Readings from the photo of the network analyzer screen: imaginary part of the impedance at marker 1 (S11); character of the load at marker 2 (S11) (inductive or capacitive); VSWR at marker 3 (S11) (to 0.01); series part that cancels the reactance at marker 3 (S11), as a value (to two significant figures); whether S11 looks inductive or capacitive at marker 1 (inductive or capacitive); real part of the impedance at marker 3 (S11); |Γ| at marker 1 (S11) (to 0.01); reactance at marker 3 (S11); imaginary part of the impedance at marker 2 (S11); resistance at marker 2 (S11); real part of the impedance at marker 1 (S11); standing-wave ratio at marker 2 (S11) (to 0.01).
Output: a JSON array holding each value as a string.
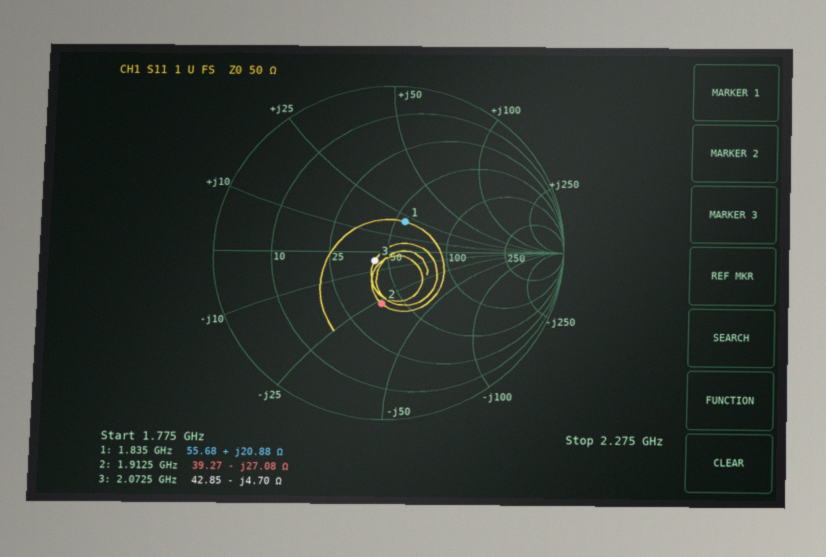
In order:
["+20.88 Ω", "capacitive", "1.20", "360 pH", "inductive", "42.85 Ω", "0.20", "-4.70 Ω", "-27.08 Ω", "39.27 Ω", "55.68 Ω", "1.91"]
